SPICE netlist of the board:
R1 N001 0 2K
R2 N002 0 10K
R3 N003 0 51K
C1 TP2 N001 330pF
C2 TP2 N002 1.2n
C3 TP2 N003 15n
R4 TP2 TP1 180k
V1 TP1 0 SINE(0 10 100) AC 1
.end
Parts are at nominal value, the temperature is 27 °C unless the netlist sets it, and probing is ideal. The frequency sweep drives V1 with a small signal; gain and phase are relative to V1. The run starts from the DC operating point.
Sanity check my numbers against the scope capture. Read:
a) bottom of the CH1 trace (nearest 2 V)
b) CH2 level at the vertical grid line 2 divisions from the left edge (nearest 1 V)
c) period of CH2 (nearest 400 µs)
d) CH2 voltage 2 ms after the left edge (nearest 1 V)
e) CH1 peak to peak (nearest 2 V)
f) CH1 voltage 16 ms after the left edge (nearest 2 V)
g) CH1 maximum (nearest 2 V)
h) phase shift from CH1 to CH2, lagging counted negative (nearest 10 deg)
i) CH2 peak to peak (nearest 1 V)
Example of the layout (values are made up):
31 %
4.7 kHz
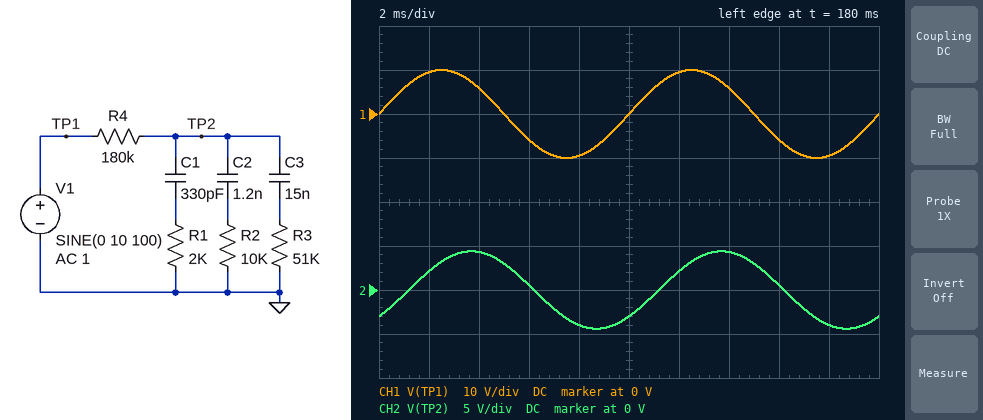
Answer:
-10 V
4 V
10.0 ms
2 V
20 V
-6 V
10 V
-40 deg
9 V
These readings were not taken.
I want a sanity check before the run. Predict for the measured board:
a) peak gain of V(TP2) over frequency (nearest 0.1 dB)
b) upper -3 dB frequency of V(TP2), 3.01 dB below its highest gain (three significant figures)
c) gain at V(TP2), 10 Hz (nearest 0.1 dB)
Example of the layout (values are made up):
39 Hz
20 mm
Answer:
0 dB
45.2 Hz
-0.2 dB
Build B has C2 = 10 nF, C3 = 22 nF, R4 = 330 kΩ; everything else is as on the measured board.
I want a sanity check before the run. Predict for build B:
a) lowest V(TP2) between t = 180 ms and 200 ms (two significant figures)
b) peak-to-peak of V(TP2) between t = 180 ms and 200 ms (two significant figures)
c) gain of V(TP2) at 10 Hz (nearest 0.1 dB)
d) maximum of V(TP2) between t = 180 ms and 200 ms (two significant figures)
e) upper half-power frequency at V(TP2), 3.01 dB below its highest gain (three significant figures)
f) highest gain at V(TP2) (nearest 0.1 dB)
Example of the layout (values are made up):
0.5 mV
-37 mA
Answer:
-1.6 V
3.3 V
-1.8 dB
1.6 V
14.0 Hz
0 dB
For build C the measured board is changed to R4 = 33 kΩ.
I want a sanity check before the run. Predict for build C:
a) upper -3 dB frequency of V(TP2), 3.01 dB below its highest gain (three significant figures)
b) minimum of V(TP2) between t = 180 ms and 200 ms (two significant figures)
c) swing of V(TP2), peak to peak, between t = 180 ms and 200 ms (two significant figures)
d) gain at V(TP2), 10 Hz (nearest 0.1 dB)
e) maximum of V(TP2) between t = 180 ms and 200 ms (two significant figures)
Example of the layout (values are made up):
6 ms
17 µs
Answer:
231 Hz
-8.6 V
17 V
0 dB
8.6 V
